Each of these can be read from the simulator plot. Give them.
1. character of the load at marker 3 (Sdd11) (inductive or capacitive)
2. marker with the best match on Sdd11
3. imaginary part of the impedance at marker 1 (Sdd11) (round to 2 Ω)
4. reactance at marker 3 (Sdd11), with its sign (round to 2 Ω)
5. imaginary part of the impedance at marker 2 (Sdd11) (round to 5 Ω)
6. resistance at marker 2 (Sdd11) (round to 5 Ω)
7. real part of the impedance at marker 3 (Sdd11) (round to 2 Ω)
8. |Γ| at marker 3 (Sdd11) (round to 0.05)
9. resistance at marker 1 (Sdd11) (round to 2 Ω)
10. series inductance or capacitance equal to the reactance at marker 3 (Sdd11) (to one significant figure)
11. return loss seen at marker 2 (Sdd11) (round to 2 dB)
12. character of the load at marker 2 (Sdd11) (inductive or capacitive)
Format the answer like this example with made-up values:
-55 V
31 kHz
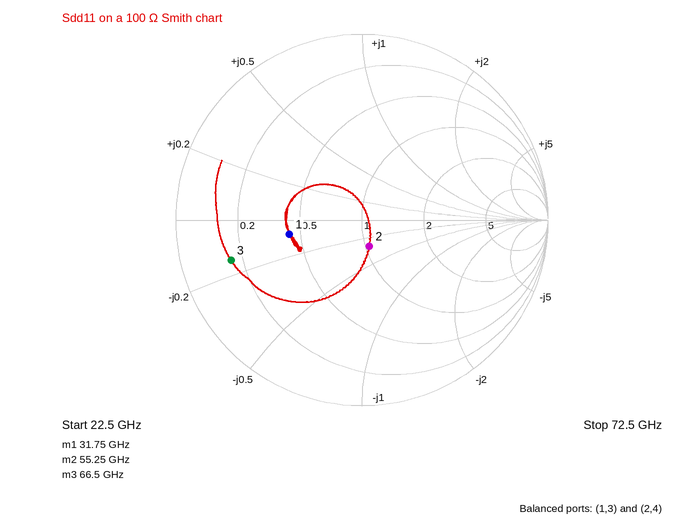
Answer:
capacitive
marker 2
-8 Ω
-14 Ω
-30 Ω
105 Ω
16 Ω
0.75
44 Ω
200 fF
16 dB
capacitive
